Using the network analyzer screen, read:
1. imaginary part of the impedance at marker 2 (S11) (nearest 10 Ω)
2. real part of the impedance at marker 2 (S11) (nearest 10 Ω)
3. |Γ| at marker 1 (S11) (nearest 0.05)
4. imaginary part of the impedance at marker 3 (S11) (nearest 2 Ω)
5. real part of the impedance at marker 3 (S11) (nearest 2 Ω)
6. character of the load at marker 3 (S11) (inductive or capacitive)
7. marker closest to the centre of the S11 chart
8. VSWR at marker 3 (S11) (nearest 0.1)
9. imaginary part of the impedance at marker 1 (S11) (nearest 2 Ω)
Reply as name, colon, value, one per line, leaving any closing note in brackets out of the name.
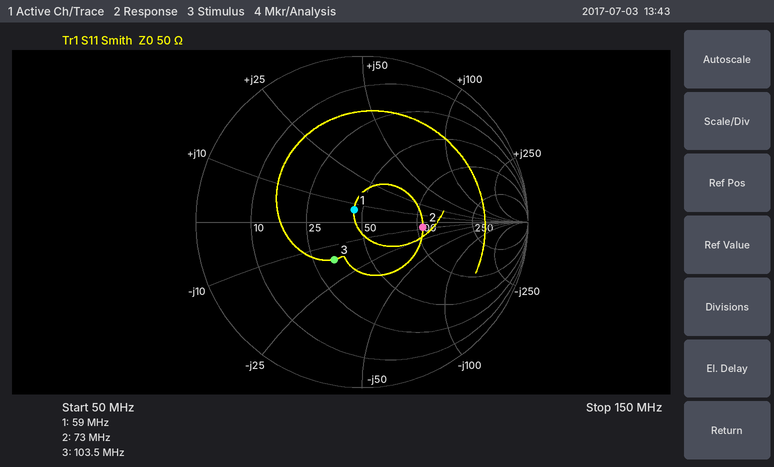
imaginary part of the impedance at marker 2 (S11): -10 Ω
real part of the impedance at marker 2 (S11): 110 Ω
|Γ| at marker 1 (S11): 0.10
imaginary part of the impedance at marker 3 (S11): -16 Ω
real part of the impedance at marker 3 (S11): 32 Ω
character of the load at marker 3 (S11): capacitive
marker closest to the centre of the S11 chart: marker 1
VSWR at marker 3 (S11): 1.8
imaginary part of the impedance at marker 1 (S11): +6 Ω
